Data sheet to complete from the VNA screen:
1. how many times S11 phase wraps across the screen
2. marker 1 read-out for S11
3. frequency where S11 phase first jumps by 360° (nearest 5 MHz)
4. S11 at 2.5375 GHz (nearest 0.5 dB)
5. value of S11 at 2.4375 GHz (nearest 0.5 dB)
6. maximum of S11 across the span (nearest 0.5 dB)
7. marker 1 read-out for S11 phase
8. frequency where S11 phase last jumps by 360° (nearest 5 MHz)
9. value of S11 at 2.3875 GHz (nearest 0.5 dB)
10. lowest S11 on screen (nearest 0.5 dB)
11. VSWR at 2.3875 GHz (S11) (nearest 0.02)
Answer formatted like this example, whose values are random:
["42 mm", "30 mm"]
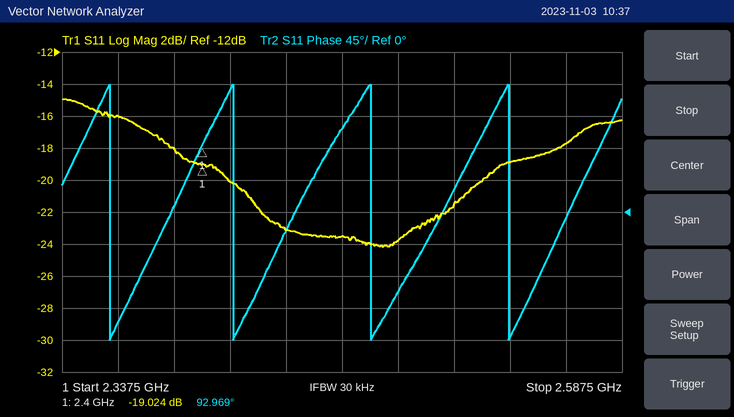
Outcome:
["4", "-19.024 dB", "2.360 GHz", "-19.0 dB", "-23.0 dB", "-15.0 dB", "92.969°", "2.535 GHz", "-18.0 dB", "-24.0 dB", "1.28"]
